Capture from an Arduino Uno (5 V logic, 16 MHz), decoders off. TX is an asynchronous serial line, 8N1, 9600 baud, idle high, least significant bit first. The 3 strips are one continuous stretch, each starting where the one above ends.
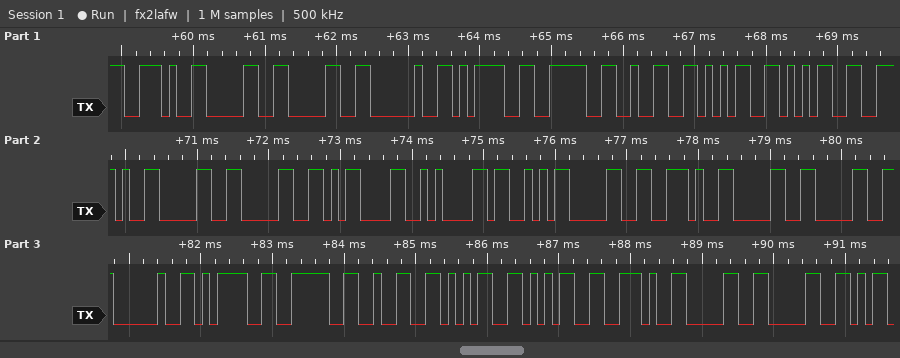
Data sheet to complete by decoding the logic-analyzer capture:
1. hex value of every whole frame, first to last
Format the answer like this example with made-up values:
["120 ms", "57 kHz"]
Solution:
["2E 30 30 20 3D 3E 32 35 35 2E 30 30 0D 0A 53 30 2E 30 30 20 3D 3E 32 35 35 2E 30 30"]
